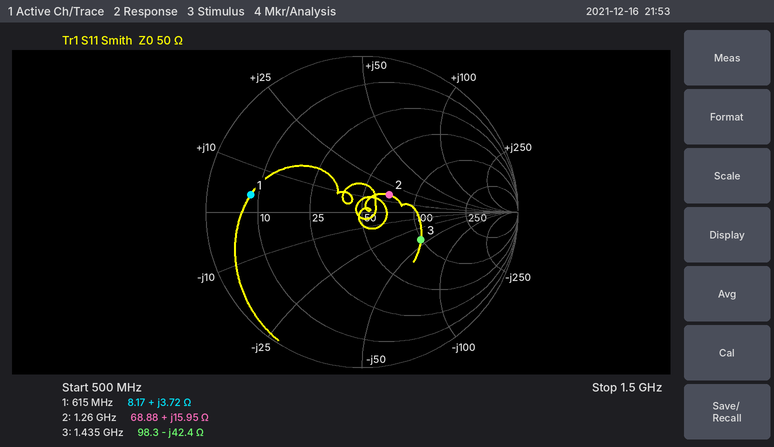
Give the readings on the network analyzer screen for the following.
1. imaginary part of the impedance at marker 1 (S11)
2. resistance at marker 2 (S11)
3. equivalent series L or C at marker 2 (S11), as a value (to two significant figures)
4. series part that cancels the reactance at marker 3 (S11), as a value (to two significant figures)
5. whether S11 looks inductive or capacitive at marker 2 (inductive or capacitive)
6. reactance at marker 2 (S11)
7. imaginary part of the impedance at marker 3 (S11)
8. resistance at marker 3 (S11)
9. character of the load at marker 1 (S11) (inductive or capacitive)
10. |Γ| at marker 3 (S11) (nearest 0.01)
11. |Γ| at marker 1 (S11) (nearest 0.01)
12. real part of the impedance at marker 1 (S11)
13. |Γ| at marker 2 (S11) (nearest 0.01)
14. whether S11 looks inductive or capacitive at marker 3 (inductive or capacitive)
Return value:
+3.72 Ω
68.88 Ω
2.0 nH
4.7 nH
inductive
+15.95 Ω
-42.4 Ω
98.3 Ω
inductive
0.42
0.72
8.17 Ω
0.21
capacitive
